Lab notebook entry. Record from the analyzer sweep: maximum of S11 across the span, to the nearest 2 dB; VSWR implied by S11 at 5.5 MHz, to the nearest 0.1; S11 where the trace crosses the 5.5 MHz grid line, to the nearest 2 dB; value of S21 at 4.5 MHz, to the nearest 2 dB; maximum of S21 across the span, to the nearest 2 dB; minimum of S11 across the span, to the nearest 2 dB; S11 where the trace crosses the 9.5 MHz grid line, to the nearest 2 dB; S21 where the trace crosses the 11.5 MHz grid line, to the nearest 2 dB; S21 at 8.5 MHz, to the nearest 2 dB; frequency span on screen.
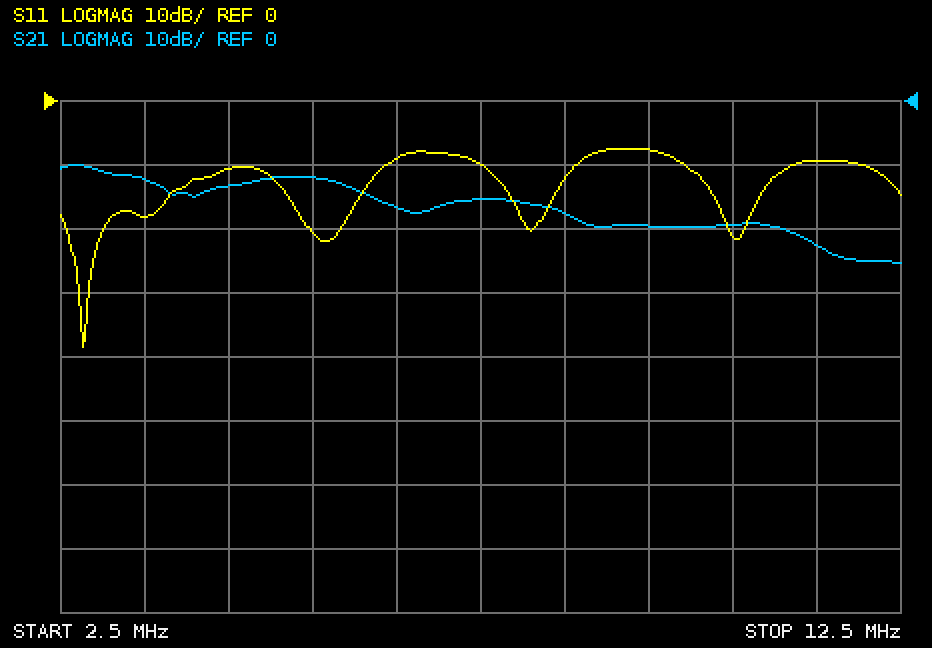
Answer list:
-8 dB
1.2
-20 dB
-14 dB
-10 dB
-38 dB
-8 dB
-22 dB
-18 dB
10 MHz
